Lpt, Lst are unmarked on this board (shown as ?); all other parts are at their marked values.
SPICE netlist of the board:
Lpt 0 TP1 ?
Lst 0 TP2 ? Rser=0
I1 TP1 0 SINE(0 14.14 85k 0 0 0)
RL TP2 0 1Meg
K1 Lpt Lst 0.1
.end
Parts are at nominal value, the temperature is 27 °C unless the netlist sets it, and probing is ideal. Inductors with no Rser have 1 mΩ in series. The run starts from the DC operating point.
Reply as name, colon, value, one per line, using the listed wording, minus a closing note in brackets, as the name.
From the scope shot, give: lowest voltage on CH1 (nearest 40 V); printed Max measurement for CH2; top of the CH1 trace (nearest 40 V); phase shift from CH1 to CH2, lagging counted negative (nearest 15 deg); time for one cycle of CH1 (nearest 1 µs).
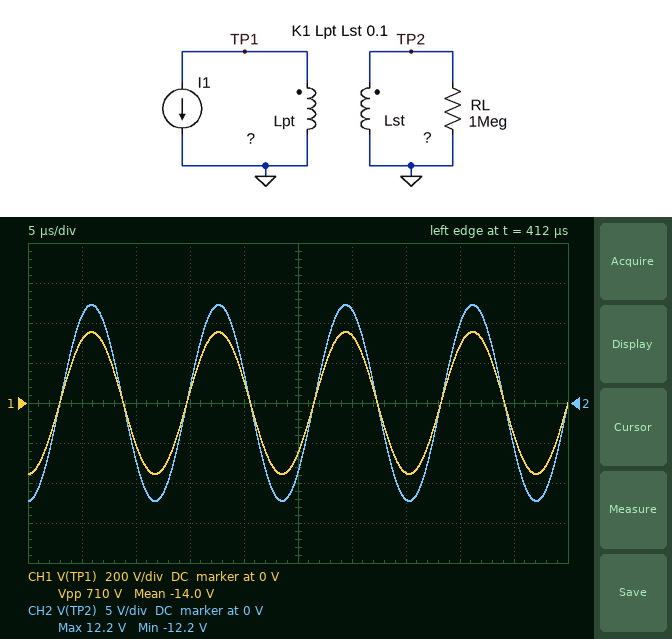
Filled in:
lowest voltage on CH1: -360 V
printed Max measurement for CH2: 12.2 V
top of the CH1 trace: 360 V
phase shift from CH1 to CH2, lagging counted negative: 0 deg
time for one cycle of CH1: 12 µs
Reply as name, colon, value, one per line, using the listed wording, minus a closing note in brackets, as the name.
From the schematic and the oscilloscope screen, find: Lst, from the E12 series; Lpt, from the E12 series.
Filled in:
Lst, from the E12 series: 5.6 µH
Lpt, from the E12 series: 47 µH
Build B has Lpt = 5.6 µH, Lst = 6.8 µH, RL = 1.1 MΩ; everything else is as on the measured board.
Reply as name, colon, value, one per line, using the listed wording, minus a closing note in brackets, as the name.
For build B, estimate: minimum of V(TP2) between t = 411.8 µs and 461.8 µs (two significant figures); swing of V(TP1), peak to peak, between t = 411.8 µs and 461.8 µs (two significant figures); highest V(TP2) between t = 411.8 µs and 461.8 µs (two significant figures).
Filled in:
minimum of V(TP2) between t = 411.8 µs and 461.8 µs: -4.7 V
swing of V(TP1), peak to peak, between t = 411.8 µs and 461.8 µs: 85 V
highest V(TP2) between t = 411.8 µs and 461.8 µs: 4.7 V
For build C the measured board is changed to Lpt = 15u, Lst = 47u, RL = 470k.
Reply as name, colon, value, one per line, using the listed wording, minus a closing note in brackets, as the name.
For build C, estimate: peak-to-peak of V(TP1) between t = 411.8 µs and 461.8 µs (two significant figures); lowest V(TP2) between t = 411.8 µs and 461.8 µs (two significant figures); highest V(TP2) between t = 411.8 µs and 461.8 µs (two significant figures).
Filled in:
peak-to-peak of V(TP1) between t = 411.8 µs and 461.8 µs: 230 V
lowest V(TP2) between t = 411.8 µs and 461.8 µs: -20 V
highest V(TP2) between t = 411.8 µs and 461.8 µs: 20 V
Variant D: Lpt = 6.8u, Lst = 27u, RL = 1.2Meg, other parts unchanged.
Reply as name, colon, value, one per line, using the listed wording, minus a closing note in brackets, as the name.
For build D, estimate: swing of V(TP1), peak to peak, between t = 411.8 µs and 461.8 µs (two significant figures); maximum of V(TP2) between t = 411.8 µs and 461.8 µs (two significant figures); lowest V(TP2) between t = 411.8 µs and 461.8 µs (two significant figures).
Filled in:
swing of V(TP1), peak to peak, between t = 411.8 µs and 461.8 µs: 100 V
maximum of V(TP2) between t = 411.8 µs and 461.8 µs: 10 V
lowest V(TP2) between t = 411.8 µs and 461.8 µs: -10 V
